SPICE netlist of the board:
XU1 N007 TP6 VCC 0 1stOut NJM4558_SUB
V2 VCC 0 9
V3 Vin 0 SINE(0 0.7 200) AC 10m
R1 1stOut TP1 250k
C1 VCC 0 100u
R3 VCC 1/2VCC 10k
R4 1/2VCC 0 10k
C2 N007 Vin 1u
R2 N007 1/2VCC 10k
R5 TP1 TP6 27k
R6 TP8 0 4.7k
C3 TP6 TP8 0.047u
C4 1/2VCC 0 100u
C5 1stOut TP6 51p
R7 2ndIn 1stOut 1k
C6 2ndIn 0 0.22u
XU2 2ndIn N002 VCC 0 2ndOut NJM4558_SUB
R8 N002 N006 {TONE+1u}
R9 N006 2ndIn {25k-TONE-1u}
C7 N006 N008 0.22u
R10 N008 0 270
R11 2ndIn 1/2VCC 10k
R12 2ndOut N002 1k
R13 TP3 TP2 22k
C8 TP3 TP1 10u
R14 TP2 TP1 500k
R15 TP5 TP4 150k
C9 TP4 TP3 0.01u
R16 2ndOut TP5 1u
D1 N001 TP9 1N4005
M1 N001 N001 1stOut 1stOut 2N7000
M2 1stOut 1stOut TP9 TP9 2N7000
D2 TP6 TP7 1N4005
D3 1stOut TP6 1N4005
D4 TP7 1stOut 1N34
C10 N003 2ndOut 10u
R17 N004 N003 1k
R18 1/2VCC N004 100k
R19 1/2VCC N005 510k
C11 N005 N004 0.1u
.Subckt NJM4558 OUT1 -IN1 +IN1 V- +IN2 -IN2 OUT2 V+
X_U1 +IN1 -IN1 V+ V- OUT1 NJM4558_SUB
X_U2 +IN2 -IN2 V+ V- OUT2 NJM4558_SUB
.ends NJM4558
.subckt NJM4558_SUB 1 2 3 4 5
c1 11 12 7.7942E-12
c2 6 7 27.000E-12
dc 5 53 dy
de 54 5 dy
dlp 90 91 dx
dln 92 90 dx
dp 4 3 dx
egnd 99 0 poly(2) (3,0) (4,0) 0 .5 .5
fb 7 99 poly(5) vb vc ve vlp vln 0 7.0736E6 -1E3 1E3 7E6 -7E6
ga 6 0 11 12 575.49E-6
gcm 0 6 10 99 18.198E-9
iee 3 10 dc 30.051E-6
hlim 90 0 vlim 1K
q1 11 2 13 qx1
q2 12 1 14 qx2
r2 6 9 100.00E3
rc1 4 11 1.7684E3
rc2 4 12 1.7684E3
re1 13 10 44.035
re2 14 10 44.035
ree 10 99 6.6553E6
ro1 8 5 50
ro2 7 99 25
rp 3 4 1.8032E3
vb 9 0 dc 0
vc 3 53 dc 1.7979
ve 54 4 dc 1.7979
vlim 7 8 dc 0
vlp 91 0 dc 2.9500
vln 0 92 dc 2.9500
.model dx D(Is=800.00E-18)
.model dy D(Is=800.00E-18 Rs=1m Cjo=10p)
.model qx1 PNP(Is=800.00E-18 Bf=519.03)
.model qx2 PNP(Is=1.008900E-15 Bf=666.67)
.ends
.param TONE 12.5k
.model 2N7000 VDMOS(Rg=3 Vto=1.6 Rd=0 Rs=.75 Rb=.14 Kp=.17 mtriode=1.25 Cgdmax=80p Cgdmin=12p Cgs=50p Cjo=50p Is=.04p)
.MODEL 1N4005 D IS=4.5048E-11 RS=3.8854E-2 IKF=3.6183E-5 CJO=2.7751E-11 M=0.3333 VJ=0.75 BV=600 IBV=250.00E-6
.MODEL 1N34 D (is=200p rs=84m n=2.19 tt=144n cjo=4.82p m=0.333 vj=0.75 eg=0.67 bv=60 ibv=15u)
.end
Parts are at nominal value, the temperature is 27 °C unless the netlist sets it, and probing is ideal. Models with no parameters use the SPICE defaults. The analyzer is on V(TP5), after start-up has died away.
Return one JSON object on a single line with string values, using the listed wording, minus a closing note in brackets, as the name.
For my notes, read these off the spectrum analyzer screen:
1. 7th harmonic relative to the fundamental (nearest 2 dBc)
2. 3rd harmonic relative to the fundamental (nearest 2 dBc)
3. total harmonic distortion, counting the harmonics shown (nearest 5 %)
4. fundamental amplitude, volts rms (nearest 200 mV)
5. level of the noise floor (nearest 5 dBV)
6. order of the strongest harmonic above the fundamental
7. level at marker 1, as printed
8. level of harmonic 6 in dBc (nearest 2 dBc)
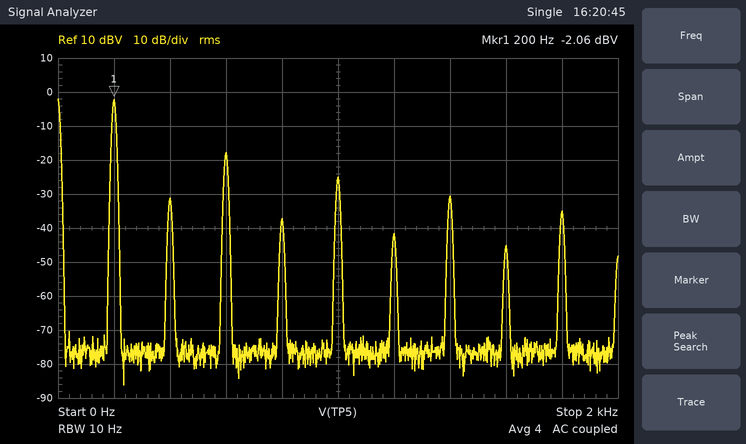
{"7th harmonic relative to the fundamental": "-28 dBc", "3rd harmonic relative to the fundamental": "-16 dBc", "total harmonic distortion, counting the harmonics shown": "20 %", "fundamental amplitude, volts rms": "800 mV", "level of the noise floor": "-75 dBV", "order of the strongest harmonic above the fundamental": "3", "level at marker 1, as printed": "-2.06 dBV", "level of harmonic 6 in dBc": "-40 dBc"}
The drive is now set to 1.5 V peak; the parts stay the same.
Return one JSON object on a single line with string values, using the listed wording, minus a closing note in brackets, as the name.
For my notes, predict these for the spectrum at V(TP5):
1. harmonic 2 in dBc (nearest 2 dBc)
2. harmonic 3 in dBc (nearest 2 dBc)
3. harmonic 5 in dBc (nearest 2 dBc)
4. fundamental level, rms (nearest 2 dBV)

{"harmonic 2 in dBc": "-34 dBc", "harmonic 3 in dBc": "-18 dBc", "harmonic 5 in dBc": "-26 dBc", "fundamental level, rms": "2 dBV"}
